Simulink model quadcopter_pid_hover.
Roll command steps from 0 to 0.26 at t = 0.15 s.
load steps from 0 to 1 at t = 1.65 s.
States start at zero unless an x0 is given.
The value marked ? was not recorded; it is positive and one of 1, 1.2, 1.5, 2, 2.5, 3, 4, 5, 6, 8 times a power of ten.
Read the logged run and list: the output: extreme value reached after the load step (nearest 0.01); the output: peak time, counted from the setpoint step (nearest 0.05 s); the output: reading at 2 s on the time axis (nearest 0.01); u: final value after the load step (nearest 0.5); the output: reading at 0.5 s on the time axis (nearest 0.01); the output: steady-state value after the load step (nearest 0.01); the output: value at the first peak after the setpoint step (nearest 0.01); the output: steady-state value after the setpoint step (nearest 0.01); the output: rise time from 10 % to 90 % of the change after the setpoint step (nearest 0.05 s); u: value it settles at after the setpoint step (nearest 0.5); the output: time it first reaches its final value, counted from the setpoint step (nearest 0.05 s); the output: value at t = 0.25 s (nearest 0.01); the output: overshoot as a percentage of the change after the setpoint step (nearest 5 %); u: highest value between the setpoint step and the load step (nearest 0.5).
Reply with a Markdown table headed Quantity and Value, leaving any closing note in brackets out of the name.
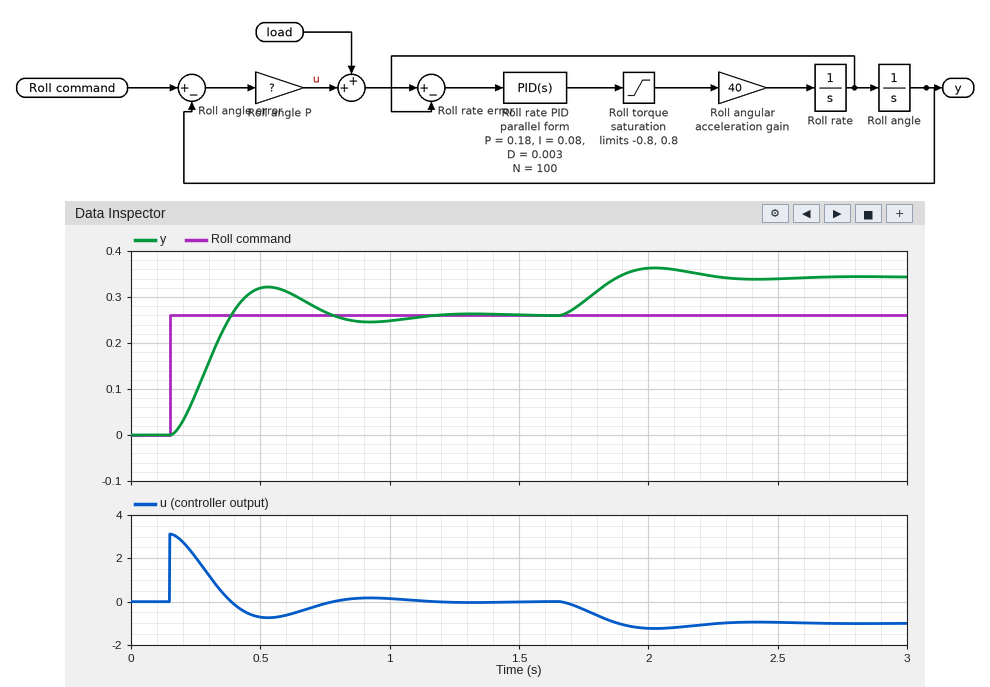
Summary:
| Quantity | Value |
|---|---|
| the output: extreme value reached after the load step | 0.36 |
| the output: peak time, counted from the setpoint step | 0.40 s |
| the output: reading at 2 s on the time axis | 0.36 |
| u: final value after the load step | -1.0 |
| the output: reading at 0.5 s on the time axis | 0.32 |
| the output: steady-state value after the load step | 0.34 |
| the output: value at the first peak after the setpoint step | 0.32 |
| the output: steady-state value after the setpoint step | 0.26 |
| the output: rise time from 10 % to 90 % of the change after the setpoint step | 0.15 s |
| u: value it settles at after the setpoint step | 0.0 |
| the output: time it first reaches its final value, counted from the setpoint step | 0.25 s |
| the output: value at t = 0.25 s | 0.09 |
| the output: overshoot as a percentage of the change after the setpoint step | 25 % |
| u: highest value between the setpoint step and the load step | 3.0 |
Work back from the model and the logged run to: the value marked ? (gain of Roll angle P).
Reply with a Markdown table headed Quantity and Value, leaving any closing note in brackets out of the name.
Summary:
| Quantity | Value |
|---|---|
| the value marked ? | 12 |
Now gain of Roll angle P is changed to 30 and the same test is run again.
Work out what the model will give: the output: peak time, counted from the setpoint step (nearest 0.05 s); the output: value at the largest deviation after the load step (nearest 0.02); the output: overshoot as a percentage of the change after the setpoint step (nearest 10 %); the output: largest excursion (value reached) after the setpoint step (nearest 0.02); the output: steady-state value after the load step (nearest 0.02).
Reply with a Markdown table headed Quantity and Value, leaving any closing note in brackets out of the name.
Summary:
| Quantity | Value |
|---|---|
| the output: peak time, counted from the setpoint step | 0.25 s |
| the output: value at the largest deviation after the load step | 0.30 |
| the output: overshoot as a percentage of the change after the setpoint step | 30 % |
| the output: largest excursion (value reached) after the setpoint step | 0.34 |
| the output: steady-state value after the load step | 0.30 |
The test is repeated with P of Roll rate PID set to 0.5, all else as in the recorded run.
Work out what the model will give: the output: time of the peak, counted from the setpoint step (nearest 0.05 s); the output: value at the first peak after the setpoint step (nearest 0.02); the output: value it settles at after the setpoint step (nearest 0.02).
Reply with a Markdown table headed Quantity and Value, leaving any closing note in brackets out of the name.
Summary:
| Quantity | Value |
|---|---|
| the output: time of the peak, counted from the setpoint step | 0.30 s |
| the output: value at the first peak after the setpoint step | 0.28 |
| the output: value it settles at after the setpoint step | 0.26 |
